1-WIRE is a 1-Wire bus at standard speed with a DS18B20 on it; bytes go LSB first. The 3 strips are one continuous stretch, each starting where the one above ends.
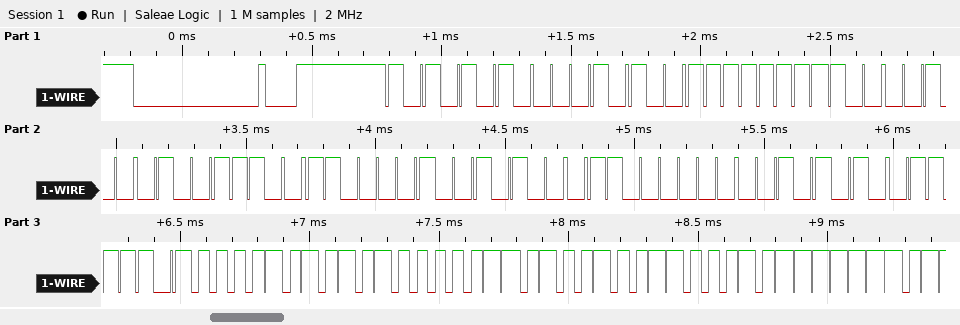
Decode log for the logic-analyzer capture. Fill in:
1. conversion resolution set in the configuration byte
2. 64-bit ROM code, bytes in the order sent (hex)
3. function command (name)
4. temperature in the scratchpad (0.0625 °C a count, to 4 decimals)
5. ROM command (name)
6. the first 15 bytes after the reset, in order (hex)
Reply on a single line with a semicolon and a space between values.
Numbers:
12 bits; 28 FF 21 72 86 14 03 54; Read Scratchpad; 85.0000 °C; Match ROM; 55 28 FF 21 72 86 14 03 54 BE 50 05 4B 46 7F
